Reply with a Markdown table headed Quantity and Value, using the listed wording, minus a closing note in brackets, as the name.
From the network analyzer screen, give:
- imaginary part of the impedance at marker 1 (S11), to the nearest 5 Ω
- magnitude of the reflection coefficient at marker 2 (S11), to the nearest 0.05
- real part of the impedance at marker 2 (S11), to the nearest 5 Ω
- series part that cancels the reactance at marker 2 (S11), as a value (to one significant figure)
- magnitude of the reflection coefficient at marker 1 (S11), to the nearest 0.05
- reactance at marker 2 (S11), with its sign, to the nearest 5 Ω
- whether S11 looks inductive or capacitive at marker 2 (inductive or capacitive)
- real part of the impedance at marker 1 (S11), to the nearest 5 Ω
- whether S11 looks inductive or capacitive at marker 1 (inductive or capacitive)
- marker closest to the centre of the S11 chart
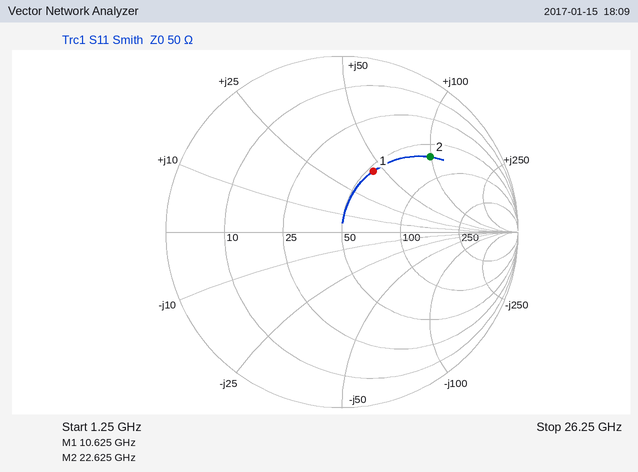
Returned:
| Quantity | Value |
|---|---|
| imaginary part of the impedance at marker 1 (S11), to the nearest 5 Ω | +45 Ω |
| magnitude of the reflection coefficient at marker 2 (S11), to the nearest 0.05 | 0.65 |
| real part of the impedance at marker 2 (S11), to the nearest 5 Ω | 65 Ω |
| series part that cancels the reactance at marker 2 (S11), as a value | 70 fF |
| magnitude of the reflection coefficient at marker 1 (S11), to the nearest 0.05 | 0.40 |
| reactance at marker 2 (S11), with its sign, to the nearest 5 Ω | +100 Ω |
| whether S11 looks inductive or capacitive at marker 2 | inductive |
| real part of the impedance at marker 1 (S11), to the nearest 5 Ω | 55 Ω |
| whether S11 looks inductive or capacitive at marker 1 | inductive |
| marker closest to the centre of the S11 chart | marker 1 |
